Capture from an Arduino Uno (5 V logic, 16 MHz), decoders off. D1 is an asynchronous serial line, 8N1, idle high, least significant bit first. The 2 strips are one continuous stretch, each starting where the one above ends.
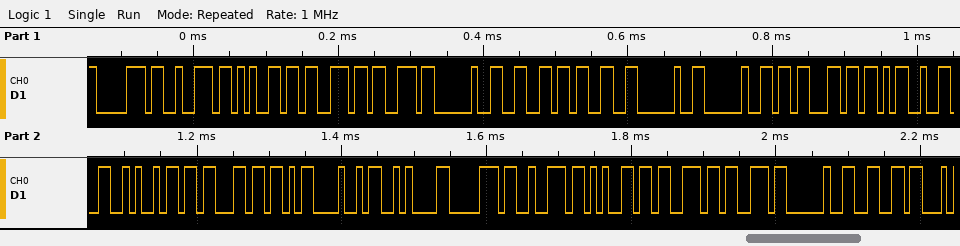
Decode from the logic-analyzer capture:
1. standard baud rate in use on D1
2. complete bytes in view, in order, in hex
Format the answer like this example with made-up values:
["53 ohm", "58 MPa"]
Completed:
["115200 baud", "70 72 65 73 73 20 66 33 20 20 1B 5B 32 4A 1B 5B 48 0A 70 72 65 73 73 20 66"]
